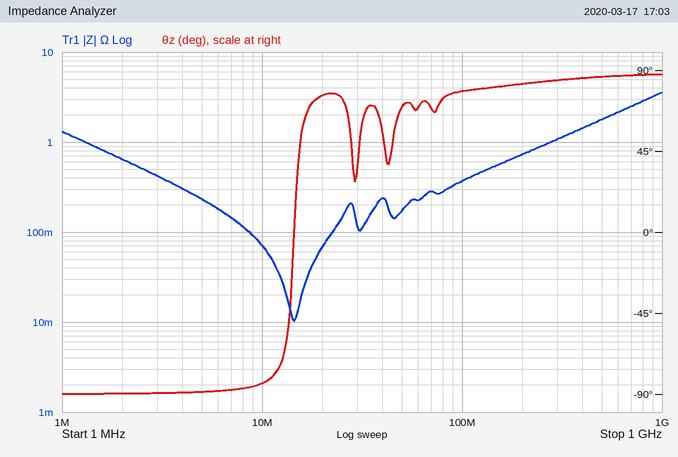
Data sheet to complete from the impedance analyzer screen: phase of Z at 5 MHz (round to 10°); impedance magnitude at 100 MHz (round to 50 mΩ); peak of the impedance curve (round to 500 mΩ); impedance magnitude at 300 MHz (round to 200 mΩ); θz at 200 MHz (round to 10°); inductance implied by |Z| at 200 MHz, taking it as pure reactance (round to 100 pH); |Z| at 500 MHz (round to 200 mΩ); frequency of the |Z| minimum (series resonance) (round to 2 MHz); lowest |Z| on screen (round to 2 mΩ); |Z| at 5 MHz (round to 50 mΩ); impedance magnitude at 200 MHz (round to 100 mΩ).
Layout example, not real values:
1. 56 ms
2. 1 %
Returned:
1. -90°
2. 350 mΩ
3. 3.5 Ω
4. 1.0 Ω
5. 80°
6. 600 pH
7. 1.8 Ω
8. 14 MHz
9. 10 mΩ
10. 250 mΩ
11. 700 mΩ
